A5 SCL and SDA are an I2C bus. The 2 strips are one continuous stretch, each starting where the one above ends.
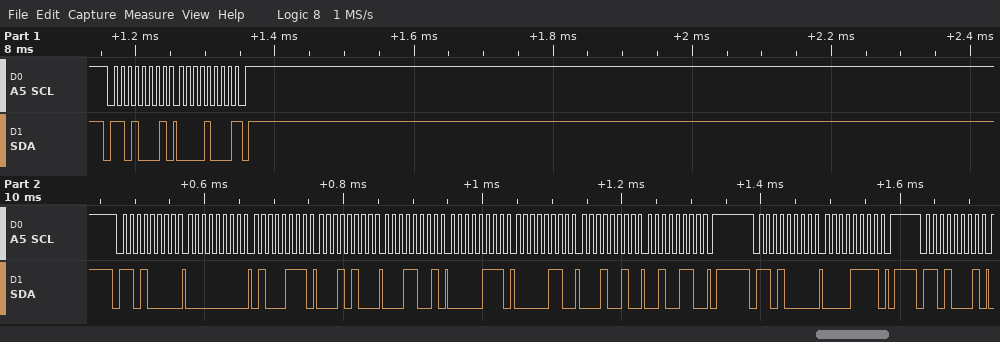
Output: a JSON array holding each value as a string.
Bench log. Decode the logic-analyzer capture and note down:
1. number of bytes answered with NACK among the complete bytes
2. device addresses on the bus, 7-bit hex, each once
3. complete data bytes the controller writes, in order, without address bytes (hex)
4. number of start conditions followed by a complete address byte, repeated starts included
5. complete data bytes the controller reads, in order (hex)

["1", "0x68", "00 47 14 19 07 06 12 26 0F", "4", "08"]
